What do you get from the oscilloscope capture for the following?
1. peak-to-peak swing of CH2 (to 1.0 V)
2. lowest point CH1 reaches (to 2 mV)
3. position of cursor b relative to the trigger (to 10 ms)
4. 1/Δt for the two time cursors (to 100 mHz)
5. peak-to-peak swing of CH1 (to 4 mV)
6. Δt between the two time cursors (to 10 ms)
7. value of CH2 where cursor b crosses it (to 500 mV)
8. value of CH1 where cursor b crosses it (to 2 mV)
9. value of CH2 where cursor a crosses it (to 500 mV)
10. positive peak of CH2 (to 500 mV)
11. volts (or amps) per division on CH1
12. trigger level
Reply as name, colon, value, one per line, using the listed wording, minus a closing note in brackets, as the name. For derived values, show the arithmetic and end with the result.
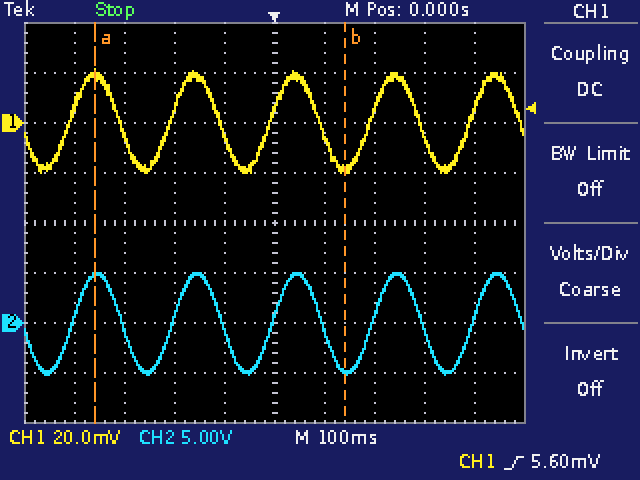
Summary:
peak-to-peak swing of CH2: 10.0 V
lowest point CH1 reaches: -20 mV
position of cursor b relative to the trigger: +140 ms
1/Δt for the two time cursors: 1 / 500 ms ≈ 2.0 Hz
peak-to-peak swing of CH1: 40 mV
Δt between the two time cursors: 500 ms
value of CH2 where cursor b crosses it: -4.5 V
value of CH1 where cursor b crosses it: -18 mV
value of CH2 where cursor a crosses it: 4.5 V
positive peak of CH2: 5.0 V
volts (or amps) per division on CH1: 20 mV
trigger level: 5.60 mV
